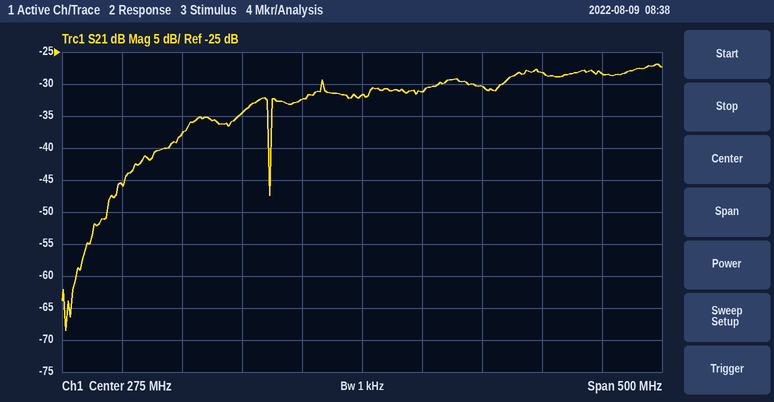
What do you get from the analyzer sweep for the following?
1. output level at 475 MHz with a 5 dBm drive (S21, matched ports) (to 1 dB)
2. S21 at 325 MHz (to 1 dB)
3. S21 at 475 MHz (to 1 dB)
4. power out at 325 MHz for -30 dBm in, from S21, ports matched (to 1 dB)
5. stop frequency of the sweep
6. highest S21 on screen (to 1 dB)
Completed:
-23 dBm
-31 dB
-28 dB
-61 dBm
525 MHz
-27 dB
